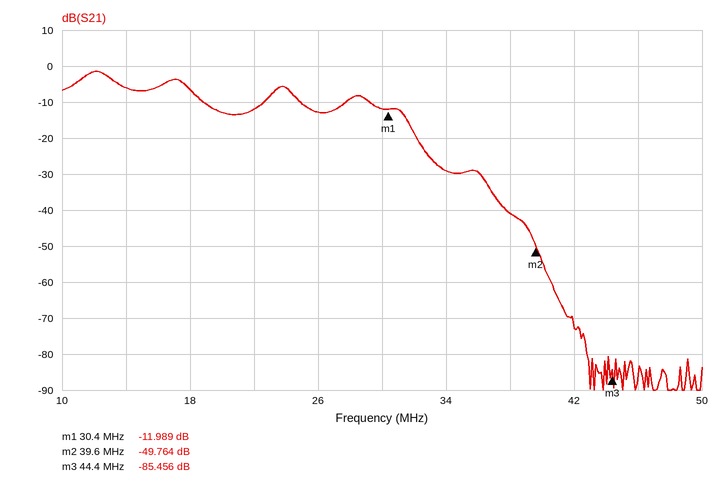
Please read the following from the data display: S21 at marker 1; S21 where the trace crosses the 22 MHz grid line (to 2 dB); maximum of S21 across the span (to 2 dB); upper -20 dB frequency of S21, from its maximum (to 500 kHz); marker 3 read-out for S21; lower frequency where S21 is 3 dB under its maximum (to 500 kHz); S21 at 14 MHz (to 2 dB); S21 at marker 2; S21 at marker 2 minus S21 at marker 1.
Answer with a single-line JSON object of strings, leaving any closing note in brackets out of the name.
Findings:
{"S21 at marker 1": "-11.989 dB", "S21 where the trace crosses the 22 MHz grid line": "-12 dB", "maximum of S21 across the span": "-2 dB", "upper -20 dB frequency of S21, from its maximum": "32.5 MHz", "marker 3 read-out for S21": "-85.456 dB", "lower frequency where S21 is 3 dB under its maximum": "11.0 MHz", "S21 at 14 MHz": "-6 dB", "S21 at marker 2": "-49.764 dB", "S21 at marker 2 minus S21 at marker 1": "-37.775 dB"}
